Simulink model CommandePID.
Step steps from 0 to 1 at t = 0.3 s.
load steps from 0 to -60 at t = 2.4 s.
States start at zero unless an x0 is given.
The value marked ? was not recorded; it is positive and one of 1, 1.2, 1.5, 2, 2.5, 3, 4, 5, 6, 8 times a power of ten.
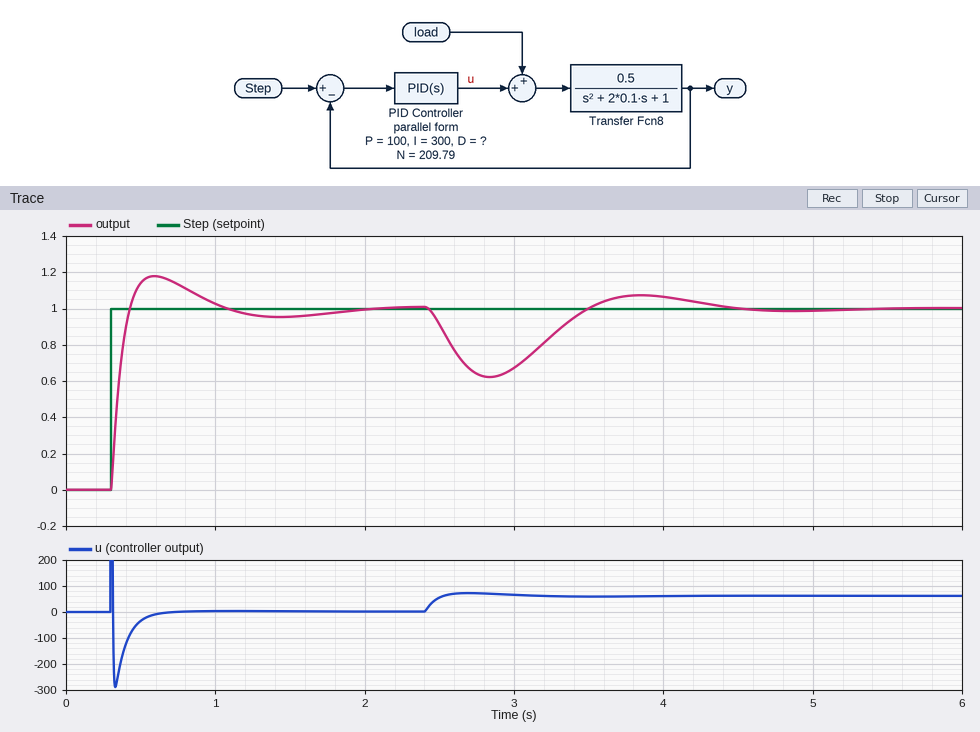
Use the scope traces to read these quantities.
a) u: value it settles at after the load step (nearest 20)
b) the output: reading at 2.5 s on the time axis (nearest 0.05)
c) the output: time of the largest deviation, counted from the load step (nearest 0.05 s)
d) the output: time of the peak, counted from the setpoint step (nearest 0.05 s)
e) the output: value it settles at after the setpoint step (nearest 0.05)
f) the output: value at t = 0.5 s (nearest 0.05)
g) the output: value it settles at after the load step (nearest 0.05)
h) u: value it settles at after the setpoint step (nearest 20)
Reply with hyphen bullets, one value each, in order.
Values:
- 60
- 0.90
- 0.45 s
- 0.30 s
- 1.00
- 1.15
- 1.00
- 0
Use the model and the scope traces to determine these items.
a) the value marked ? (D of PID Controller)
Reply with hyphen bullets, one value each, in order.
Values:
- 30
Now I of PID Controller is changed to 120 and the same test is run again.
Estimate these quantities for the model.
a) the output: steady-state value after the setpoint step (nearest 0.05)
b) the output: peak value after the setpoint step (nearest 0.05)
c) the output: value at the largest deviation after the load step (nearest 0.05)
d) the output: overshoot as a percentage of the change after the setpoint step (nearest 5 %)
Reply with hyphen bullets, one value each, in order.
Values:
- 1.00
- 1.15
- 0.55
- 15 %
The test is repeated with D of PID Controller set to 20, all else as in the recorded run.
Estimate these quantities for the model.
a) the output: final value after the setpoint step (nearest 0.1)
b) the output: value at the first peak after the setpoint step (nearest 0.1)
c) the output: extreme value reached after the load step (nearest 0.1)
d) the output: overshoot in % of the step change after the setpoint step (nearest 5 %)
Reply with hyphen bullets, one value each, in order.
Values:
- 1.0
- 1.3
- 0.5
- 30 %
